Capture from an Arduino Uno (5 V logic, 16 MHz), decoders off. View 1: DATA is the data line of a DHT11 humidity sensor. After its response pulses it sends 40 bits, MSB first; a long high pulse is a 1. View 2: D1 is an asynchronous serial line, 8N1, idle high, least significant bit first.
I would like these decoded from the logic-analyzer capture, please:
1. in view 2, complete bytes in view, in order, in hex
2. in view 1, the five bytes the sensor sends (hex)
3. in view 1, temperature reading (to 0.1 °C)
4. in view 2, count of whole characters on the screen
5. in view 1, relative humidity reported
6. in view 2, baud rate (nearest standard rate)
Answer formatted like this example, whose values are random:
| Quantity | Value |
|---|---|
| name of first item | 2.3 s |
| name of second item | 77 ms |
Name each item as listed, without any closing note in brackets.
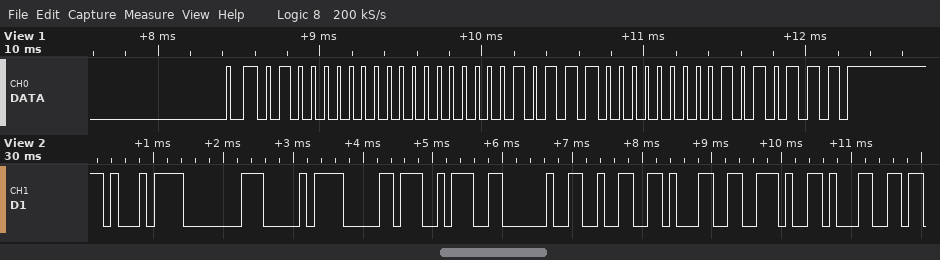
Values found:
| Quantity | Value |
|---|---|
| in view 2, complete bytes in view, in order, in hex | 0xD1 0x80 0xD0 0xB0 0x3A 0x20 0x32 0x31 0x2E 0x31 |
| in view 1, the five bytes the sensor sends | 40 00 17 00 57 |
| in view 1, temperature reading | 23.0 °C |
| in view 2, count of whole characters on the screen | 10 |
| in view 1, relative humidity reported | 64 % |
| in view 2, baud rate | 9600 baud |
